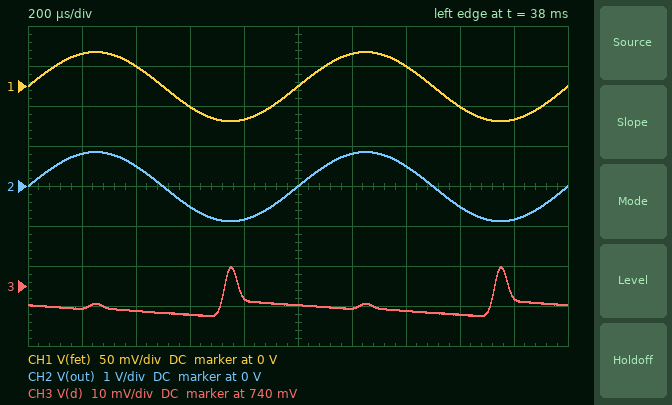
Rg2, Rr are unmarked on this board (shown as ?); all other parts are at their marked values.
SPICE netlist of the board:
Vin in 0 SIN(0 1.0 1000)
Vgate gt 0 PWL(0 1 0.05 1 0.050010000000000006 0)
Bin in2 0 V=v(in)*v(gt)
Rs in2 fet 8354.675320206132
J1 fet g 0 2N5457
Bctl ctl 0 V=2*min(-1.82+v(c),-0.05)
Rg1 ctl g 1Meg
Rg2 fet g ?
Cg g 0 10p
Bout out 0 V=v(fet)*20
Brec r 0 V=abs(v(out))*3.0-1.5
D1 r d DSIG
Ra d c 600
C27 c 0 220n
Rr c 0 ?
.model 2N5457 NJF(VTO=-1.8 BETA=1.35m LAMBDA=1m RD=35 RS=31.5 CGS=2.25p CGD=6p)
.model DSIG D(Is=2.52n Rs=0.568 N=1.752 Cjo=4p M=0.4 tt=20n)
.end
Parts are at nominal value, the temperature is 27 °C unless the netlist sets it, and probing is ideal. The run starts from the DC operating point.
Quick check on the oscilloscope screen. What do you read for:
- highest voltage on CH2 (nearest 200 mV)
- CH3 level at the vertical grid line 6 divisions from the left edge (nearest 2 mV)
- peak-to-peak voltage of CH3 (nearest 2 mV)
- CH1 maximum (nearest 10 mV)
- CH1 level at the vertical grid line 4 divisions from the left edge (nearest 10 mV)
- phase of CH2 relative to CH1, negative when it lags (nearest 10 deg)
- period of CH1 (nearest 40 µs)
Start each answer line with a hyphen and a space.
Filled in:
- 800 mV
- 734 mV
- 12 mV
- 40 mV
- -40 mV
- 0 deg
- 1.00 ms
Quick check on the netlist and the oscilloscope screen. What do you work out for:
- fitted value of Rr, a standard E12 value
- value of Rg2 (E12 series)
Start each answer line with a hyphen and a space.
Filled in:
- 680 kΩ
- 390 kΩ
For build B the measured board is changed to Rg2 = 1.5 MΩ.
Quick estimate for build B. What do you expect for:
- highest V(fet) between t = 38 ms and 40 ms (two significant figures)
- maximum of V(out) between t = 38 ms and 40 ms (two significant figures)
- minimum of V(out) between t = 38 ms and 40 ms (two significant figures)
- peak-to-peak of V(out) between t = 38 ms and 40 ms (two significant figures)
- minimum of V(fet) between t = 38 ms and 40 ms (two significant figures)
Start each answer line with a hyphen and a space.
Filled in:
- 51 mV
- 1.0 V
- -1.0 V
- 2.0 V
- -51 mV
